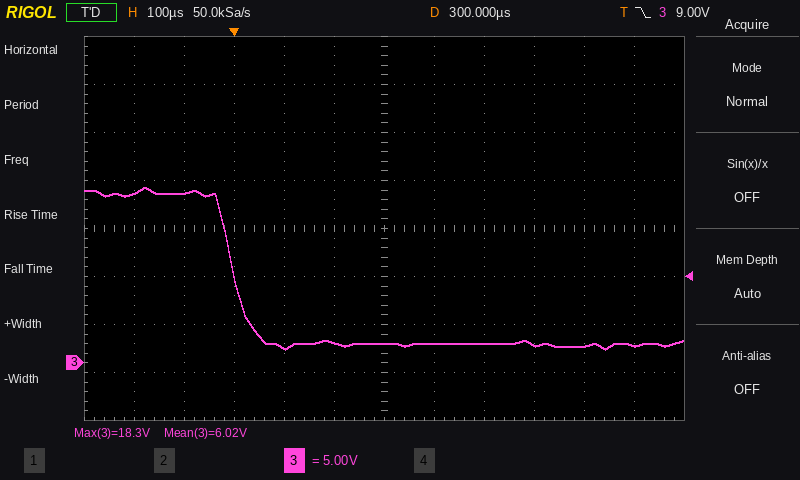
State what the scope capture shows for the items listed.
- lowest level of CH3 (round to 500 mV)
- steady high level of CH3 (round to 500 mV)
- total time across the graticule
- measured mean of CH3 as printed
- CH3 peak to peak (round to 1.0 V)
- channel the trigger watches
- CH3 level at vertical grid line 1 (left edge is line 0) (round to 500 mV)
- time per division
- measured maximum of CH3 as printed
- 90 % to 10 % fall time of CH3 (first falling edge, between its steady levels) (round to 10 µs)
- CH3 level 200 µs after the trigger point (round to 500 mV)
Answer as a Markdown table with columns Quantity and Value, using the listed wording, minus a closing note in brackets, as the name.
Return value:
| Quantity | Value |
|---|---|
| lowest level of CH3 | 1.5 V |
| steady high level of CH3 | 17.5 V |
| total time across the graticule | 1.2 ms |
| measured mean of CH3 as printed | 6.02 V |
| CH3 peak to peak | 17.0 V |
| channel the trigger watches | CH3 |
| CH3 level at vertical grid line 1 (left edge is line 0) | 17.5 V |
| time per division | 100 µs |
| measured maximum of CH3 as printed | 18.3 V |
| 90 % to 10 % fall time of CH3 (first falling edge, between its steady levels) | 70 µs |
| CH3 level 200 µs after the trigger point | 2.0 V |
